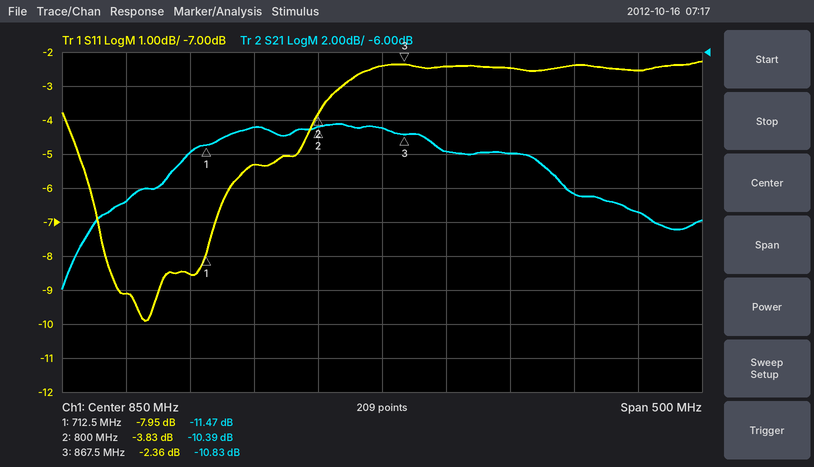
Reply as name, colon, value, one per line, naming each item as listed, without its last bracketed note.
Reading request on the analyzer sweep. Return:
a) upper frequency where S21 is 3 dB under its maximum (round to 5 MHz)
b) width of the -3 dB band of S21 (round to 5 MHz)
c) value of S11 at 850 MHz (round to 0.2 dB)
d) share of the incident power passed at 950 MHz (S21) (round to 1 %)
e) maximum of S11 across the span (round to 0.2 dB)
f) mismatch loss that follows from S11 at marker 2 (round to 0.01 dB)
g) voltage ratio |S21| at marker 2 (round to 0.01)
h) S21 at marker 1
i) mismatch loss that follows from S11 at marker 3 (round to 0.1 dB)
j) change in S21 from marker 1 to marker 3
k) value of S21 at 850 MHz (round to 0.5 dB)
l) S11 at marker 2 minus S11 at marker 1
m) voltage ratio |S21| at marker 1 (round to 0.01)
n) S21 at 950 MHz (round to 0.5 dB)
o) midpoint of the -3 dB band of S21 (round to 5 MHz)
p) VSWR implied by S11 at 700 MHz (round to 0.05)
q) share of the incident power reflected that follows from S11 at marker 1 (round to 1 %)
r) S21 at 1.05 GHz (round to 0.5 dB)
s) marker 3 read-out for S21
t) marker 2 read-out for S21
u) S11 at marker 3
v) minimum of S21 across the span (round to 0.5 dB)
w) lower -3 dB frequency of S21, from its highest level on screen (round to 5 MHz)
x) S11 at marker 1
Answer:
upper frequency where S21 is 3 dB under its maximum: 985 MHz
width of the -3 dB band of S21: 300 MHz
value of S11 at 850 MHz: -2.4 dB
share of the incident power passed at 950 MHz (S21): 6 %
maximum of S11 across the span: -2.2 dB
mismatch loss that follows from S11 at marker 2: 2.32 dB
voltage ratio |S21| at marker 2: 0.30
S21 at marker 1: -11.47 dB
mismatch loss that follows from S11 at marker 3: 3.8 dB
change in S21 from marker 1 to marker 3: 0.64 dB
value of S21 at 850 MHz: -10.5 dB
S11 at marker 2 minus S11 at marker 1: 4.12 dB
voltage ratio |S21| at marker 1: 0.27
S21 at 950 MHz: -12.0 dB
midpoint of the -3 dB band of S21: 835 MHz
VSWR implied by S11 at 700 MHz: 2.20
share of the incident power reflected that follows from S11 at marker 1: 16 %
S21 at 1.05 GHz: -15.5 dB
marker 3 read-out for S21: -10.83 dB
marker 2 read-out for S21: -10.39 dB
S11 at marker 3: -2.36 dB
minimum of S21 across the span: -20.0 dB
lower -3 dB frequency of S21, from its highest level on screen: 685 MHz
S11 at marker 1: -7.95 dB
